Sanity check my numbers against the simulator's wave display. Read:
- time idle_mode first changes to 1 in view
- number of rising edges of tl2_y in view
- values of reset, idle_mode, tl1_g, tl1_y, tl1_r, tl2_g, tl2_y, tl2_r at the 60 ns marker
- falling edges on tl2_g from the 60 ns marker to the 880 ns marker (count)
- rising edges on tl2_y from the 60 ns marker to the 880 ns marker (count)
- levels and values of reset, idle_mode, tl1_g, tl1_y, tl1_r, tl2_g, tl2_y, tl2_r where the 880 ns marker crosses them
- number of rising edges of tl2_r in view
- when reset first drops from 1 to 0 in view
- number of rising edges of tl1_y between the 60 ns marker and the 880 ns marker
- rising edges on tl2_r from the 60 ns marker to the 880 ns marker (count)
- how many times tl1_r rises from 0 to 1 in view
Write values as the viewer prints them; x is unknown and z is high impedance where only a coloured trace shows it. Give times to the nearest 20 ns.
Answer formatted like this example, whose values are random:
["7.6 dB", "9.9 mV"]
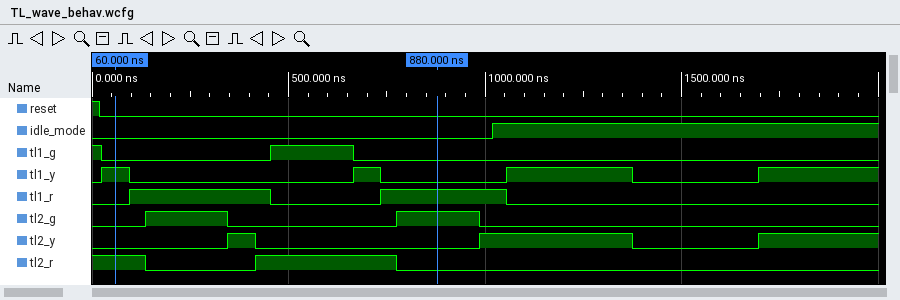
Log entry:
["1020 ns", "3", "reset=0, idle_mode=0, tl1_g=0, tl1_y=1, tl1_r=0, tl2_g=0, tl2_y=0, tl2_r=1", "1", "1", "reset=0, idle_mode=0, tl1_g=0, tl1_y=0, tl1_r=1, tl2_g=1, tl2_y=0, tl2_r=0", "1", "20 ns", "1", "1", "2"]
